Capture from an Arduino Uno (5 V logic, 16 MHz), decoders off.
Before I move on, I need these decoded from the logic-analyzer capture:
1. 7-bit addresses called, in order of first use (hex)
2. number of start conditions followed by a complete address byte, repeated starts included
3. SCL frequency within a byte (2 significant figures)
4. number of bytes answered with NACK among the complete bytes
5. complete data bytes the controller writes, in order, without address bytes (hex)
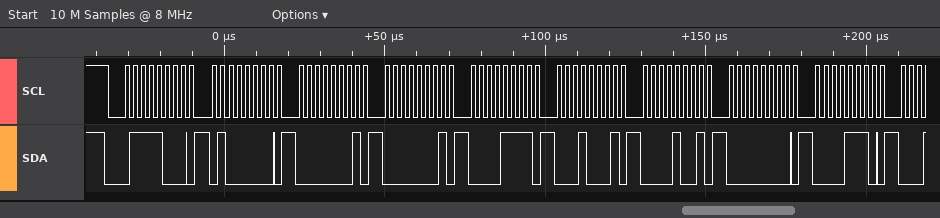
0x3C
1
400 kHz
0
40 01 01 0F 11 09 00 0E
